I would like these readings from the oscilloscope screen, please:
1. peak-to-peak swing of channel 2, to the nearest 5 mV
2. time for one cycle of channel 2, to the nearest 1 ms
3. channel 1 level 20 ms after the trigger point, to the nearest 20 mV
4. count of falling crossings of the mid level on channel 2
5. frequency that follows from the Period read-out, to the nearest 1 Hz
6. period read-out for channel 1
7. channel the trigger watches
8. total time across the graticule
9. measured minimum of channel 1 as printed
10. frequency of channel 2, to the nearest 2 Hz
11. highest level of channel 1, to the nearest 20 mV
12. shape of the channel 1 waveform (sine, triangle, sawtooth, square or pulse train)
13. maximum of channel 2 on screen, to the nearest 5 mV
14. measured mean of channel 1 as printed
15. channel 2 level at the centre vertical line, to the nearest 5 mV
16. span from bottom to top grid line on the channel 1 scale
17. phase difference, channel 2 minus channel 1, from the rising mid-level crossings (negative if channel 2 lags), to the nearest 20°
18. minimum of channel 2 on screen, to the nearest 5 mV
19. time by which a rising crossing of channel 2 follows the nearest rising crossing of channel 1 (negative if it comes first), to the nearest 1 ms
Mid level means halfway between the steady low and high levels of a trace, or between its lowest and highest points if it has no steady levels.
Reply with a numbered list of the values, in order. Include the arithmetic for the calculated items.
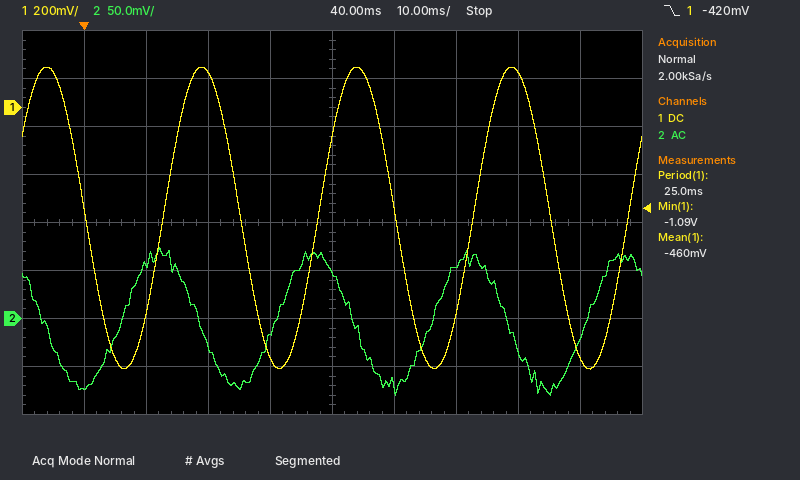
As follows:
1. 75 mV − (-80 mV) = 155 mV
2. 25 ms
3. 140 mV
4. 4
5. 1 / 25.0 ms ≈ 40 Hz
6. 25.0 ms
7. channel 1
8. 100 ms
9. -1.09 V
10. 1 / 25 ms ≈ 40 Hz
11. 160 mV
12. sine
13. 75 mV
14. -460 mV
15. 50 mV
16. 1.6 V
17. −360° × (-7 ms) / 25 ms ≈ +101°, so +100° to the nearest 20°
18. -80 mV
19. -7 ms
